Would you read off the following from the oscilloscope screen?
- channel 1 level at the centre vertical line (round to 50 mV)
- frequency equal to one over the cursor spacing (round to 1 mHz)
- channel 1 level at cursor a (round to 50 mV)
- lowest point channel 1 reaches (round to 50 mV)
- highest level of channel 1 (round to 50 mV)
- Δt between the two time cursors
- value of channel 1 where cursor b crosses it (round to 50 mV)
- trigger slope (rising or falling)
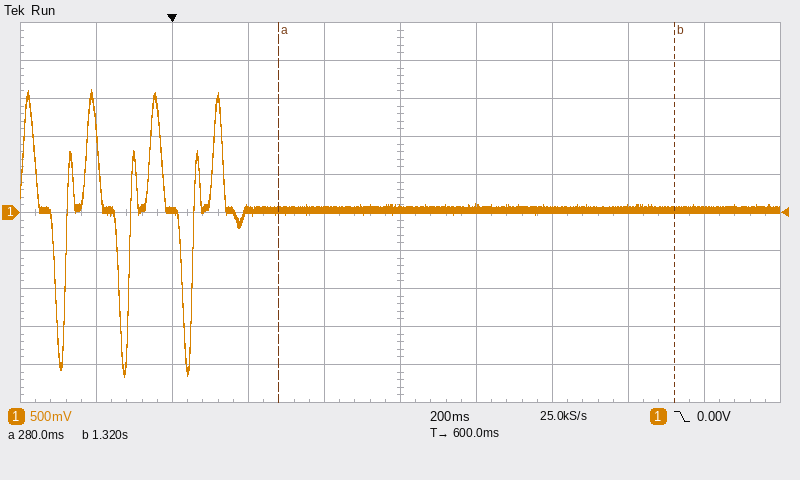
50 mV
962 mHz
50 mV
-2.15 V
1.60 V
1.04 s
50 mV
falling
